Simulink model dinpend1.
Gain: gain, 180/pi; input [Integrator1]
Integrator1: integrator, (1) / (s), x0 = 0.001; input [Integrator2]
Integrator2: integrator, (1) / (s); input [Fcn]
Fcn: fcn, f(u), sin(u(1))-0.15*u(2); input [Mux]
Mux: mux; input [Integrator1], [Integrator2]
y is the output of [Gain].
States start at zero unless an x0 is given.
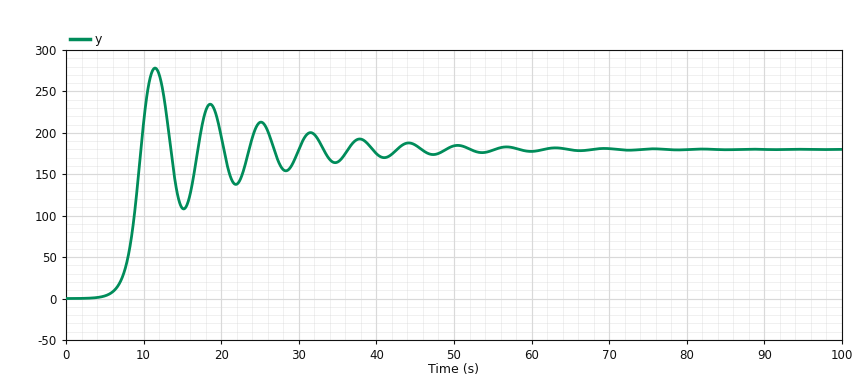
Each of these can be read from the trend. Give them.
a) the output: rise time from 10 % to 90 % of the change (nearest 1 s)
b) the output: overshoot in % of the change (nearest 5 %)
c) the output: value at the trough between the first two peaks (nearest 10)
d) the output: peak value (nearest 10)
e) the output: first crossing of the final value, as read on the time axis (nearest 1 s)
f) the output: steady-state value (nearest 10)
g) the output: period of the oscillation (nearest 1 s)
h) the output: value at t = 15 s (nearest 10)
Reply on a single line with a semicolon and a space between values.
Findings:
3 s; 55 %; 110; 280; 10 s; 180; 7 s; 110
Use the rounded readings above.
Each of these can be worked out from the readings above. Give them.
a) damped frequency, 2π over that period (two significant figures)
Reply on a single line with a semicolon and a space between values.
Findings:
0.90 rad/s
